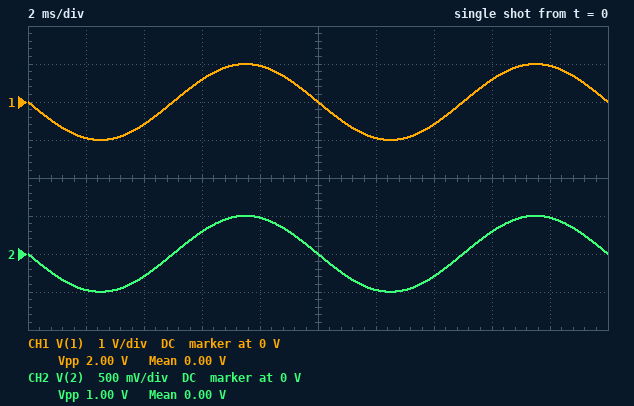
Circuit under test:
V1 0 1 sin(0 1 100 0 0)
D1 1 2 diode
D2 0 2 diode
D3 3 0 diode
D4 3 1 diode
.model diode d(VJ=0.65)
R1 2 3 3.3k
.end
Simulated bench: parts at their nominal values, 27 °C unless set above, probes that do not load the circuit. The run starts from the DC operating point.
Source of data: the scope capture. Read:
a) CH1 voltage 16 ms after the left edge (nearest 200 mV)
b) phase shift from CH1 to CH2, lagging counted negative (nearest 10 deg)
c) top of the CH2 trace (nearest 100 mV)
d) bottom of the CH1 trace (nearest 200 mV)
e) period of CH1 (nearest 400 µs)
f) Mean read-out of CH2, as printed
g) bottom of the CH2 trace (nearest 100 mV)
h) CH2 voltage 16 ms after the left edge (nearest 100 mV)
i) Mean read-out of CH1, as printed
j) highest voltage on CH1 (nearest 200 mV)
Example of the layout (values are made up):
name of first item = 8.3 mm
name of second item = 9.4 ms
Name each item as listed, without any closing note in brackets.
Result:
CH1 voltage 16 ms after the left edge = 600 mV
phase shift from CH1 to CH2, lagging counted negative = 0 deg
top of the CH2 trace = 500 mV
bottom of the CH1 trace = -1.0 V
period of CH1 = 10.0 ms
Mean read-out of CH2, as printed = 0.00 V
bottom of the CH2 trace = -500 mV
CH2 voltage 16 ms after the left edge = 300 mV
Mean read-out of CH1, as printed = 0.00 V
highest voltage on CH1 = 1.0 V
